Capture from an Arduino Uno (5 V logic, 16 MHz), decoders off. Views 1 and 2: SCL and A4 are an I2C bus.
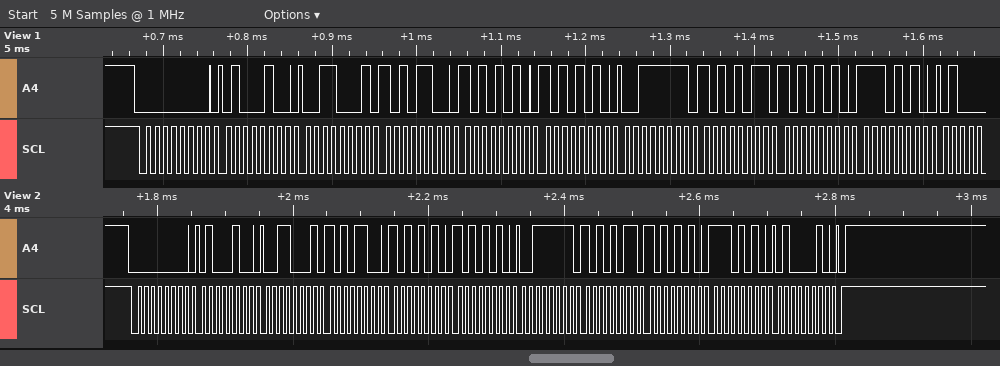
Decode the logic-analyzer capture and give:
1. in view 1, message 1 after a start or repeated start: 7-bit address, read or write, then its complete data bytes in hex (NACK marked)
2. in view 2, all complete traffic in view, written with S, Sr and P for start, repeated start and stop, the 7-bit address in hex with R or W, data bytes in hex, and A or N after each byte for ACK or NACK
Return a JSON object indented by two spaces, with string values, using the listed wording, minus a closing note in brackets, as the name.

{
  "in view 1, message 1 after a start or repeated start: 7-bit address, read or write, then its complete data bytes in hex": "0x00 write: 44 31 AC AA AA 3F AB AA EA",
  "in view 2, all complete traffic in view, written with S, Sr and P for start, repeated start and stop, the 7-bit address in hex with R or W, data bytes in hex, and A or N after each byte for ACK or NACK": "S 00W A 44 A 31 A AC A AA A AA A 3F A AB A AA A EA A 42 A P"
}
